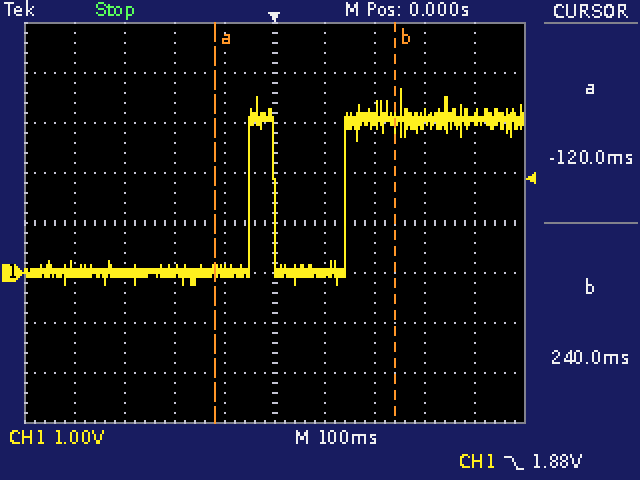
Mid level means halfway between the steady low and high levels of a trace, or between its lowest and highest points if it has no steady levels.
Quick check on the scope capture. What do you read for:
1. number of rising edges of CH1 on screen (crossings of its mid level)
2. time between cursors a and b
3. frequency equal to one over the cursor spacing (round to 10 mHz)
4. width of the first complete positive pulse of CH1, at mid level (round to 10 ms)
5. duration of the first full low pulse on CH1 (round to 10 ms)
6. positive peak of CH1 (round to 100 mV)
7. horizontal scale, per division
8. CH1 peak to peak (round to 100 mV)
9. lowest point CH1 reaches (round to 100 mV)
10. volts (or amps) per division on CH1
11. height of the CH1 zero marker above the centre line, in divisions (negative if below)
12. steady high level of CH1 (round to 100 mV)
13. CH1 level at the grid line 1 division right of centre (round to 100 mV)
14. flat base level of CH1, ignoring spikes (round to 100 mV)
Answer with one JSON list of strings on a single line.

["2", "360 ms", "2.78 Hz", "50 ms", "140 ms", "3.7 V", "100 ms", "3.9 V", "-200 mV", "1 V", "-1.0 div", "3.1 V", "0.0 V", "0.0 V"]
